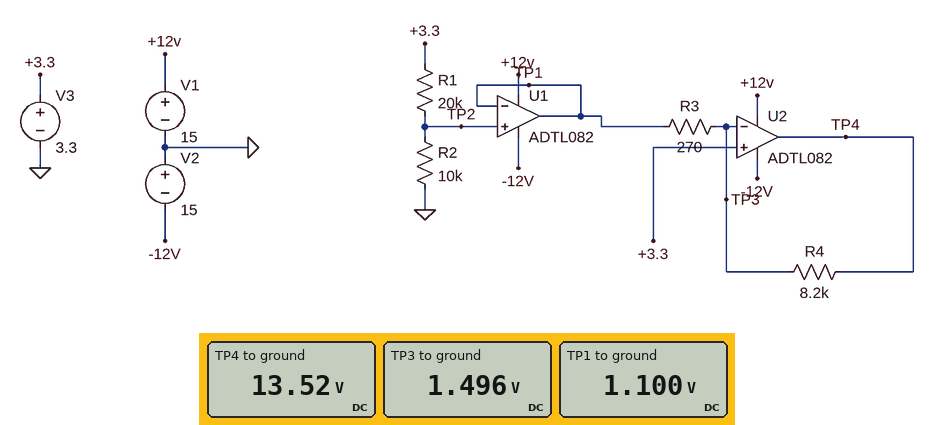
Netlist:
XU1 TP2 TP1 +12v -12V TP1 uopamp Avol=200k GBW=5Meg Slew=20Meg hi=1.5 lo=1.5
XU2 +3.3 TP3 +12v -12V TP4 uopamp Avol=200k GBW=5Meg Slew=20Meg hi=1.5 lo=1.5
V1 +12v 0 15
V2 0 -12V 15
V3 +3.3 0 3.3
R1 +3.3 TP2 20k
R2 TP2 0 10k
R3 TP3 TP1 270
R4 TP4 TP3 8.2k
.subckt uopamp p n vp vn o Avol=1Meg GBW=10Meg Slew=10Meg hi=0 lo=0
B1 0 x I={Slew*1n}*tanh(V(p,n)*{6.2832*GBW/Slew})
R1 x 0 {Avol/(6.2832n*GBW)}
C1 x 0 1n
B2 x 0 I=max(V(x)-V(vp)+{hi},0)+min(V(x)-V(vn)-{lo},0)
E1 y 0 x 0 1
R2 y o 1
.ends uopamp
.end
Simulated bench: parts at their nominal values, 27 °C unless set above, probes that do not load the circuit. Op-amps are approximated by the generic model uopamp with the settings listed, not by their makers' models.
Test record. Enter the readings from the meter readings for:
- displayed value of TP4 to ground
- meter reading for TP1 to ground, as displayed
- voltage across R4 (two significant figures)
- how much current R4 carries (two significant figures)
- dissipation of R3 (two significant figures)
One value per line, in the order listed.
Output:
13.52 V
1.100 V
12 V
1.5 mA
580 µW
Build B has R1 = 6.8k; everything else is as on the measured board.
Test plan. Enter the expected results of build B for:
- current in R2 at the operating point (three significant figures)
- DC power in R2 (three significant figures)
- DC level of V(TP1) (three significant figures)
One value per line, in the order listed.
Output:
196 µA
386 µW
1.96 V
